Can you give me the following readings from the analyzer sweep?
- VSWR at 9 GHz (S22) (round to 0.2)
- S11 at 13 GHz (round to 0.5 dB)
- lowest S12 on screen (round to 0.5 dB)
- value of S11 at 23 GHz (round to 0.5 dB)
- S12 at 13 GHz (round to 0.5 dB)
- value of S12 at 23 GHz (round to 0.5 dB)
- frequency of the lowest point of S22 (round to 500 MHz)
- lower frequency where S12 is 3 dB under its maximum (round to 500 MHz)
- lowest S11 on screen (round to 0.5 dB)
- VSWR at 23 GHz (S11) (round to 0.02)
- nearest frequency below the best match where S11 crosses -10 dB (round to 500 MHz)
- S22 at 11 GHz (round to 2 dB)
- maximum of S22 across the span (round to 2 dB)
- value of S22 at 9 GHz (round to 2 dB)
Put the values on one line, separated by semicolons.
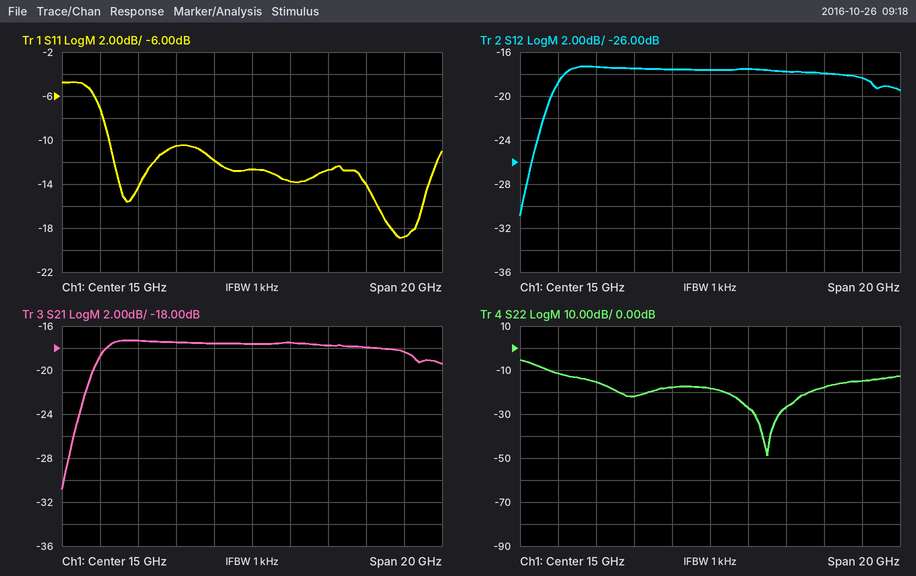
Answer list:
1.4; -12.0 dB; -31.0 dB; -19.0 dB; -17.5 dB; -18.5 dB; 18.0 GHz; 6.5 GHz; -19.0 dB; 1.26; 7.5 GHz; -22 dB; -6 dB; -16 dB
